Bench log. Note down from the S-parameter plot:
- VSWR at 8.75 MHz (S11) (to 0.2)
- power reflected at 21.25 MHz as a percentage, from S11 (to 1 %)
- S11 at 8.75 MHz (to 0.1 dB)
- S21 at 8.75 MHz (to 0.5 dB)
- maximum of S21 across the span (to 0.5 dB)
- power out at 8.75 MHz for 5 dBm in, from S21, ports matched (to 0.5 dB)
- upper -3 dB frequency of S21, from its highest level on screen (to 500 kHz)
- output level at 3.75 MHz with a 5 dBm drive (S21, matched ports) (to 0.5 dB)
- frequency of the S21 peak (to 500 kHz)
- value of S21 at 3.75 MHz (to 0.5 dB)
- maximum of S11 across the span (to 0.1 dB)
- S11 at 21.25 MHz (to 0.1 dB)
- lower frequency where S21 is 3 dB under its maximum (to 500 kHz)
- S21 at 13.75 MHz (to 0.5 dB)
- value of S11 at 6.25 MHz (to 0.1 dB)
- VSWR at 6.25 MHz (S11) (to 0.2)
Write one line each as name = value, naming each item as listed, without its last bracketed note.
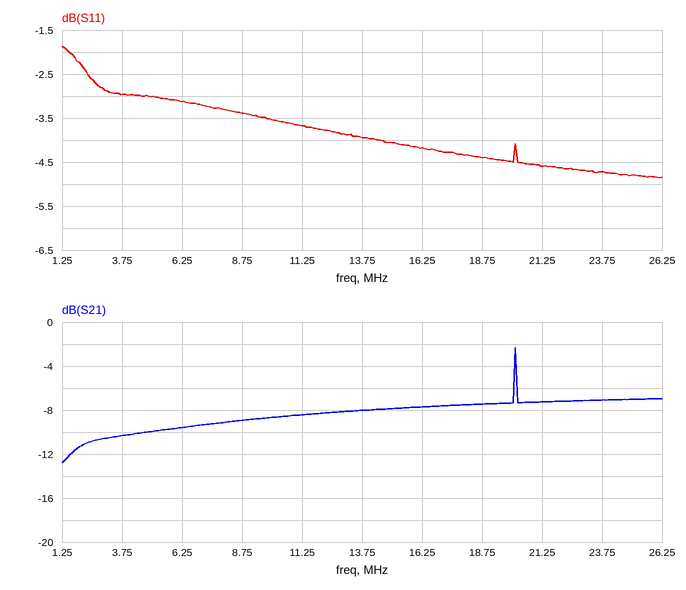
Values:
VSWR at 8.75 MHz (S11) = 5.2
power reflected at 21.25 MHz as a percentage, from S11 = 35 %
S11 at 8.75 MHz = -3.4 dB
S21 at 8.75 MHz = -9.0 dB
maximum of S21 across the span = -2.5 dB
power out at 8.75 MHz for 5 dBm in, from S21, ports matched = -4.0 dBm
upper -3 dB frequency of S21, from its highest level on screen = 20.0 MHz
output level at 3.75 MHz with a 5 dBm drive (S21, matched ports) = -5.5 dBm
frequency of the S21 peak = 20.0 MHz
value of S21 at 3.75 MHz = -10.5 dB
maximum of S11 across the span = -1.9 dB
S11 at 21.25 MHz = -4.6 dB
lower frequency where S21 is 3 dB under its maximum = 20.0 MHz
S21 at 13.75 MHz = -8.0 dB
value of S11 at 6.25 MHz = -3.1 dB
VSWR at 6.25 MHz (S11) = 5.6
